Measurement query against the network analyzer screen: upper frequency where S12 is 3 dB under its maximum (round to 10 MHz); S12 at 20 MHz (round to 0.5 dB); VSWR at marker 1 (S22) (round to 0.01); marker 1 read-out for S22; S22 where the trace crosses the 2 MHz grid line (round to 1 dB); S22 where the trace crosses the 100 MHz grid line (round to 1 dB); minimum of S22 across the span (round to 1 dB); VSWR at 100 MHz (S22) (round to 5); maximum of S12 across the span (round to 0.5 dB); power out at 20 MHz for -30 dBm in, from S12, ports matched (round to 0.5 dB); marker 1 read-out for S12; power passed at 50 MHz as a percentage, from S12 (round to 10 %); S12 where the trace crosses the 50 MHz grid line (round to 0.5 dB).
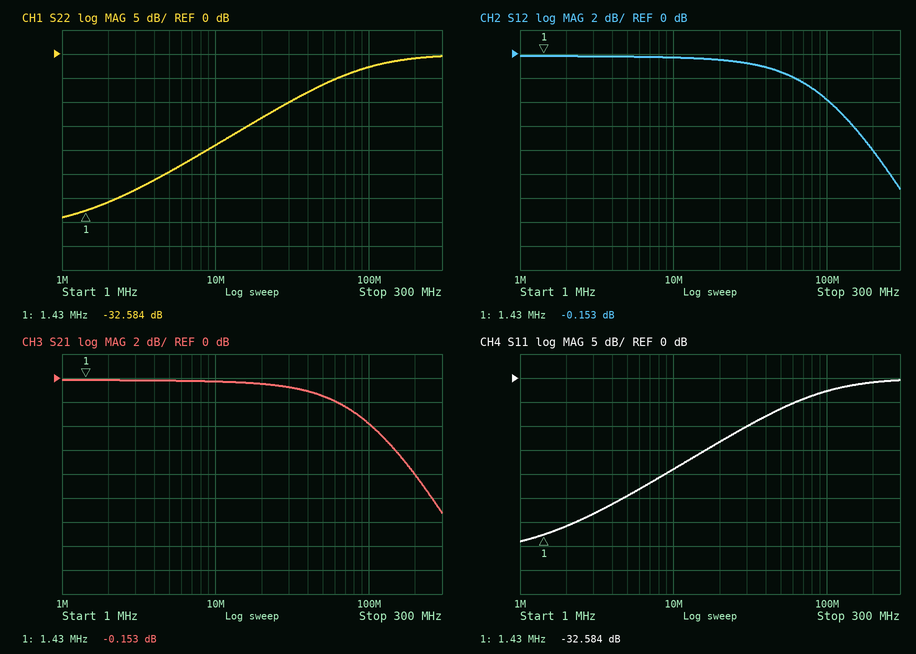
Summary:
90 MHz
-0.5 dB
1.05
-32.584 dB
-31 dB
-3 dB
-34 dB
5
0.0 dB
-30.5 dBm
-0.153 dB
70 %
-1.5 dB
